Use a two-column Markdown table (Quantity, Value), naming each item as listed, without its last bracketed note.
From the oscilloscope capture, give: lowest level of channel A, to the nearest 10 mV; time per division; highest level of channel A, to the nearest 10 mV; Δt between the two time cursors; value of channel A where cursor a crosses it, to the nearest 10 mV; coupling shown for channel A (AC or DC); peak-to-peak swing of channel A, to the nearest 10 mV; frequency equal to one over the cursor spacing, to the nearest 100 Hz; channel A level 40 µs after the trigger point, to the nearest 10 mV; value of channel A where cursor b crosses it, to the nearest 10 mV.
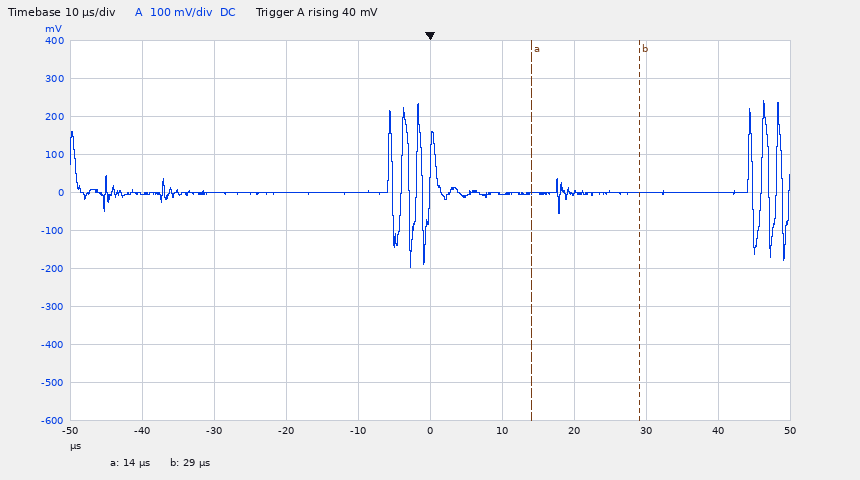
| Quantity | Value |
|---|---|
| lowest level of channel A, to the nearest 10 mV | -200 mV |
| time per division | 10 µs |
| highest level of channel A, to the nearest 10 mV | 240 mV |
| Δt between the two time cursors | 15 µs |
| value of channel A where cursor a crosses it, to the nearest 10 mV | 0 mV |
| coupling shown for channel A | DC |
| peak-to-peak swing of channel A, to the nearest 10 mV | 440 mV |
| frequency equal to one over the cursor spacing, to the nearest 100 Hz | 66.7 kHz |
| channel A level 40 µs after the trigger point, to the nearest 10 mV | 0 mV |
| value of channel A where cursor b crosses it, to the nearest 10 mV | 0 mV |
